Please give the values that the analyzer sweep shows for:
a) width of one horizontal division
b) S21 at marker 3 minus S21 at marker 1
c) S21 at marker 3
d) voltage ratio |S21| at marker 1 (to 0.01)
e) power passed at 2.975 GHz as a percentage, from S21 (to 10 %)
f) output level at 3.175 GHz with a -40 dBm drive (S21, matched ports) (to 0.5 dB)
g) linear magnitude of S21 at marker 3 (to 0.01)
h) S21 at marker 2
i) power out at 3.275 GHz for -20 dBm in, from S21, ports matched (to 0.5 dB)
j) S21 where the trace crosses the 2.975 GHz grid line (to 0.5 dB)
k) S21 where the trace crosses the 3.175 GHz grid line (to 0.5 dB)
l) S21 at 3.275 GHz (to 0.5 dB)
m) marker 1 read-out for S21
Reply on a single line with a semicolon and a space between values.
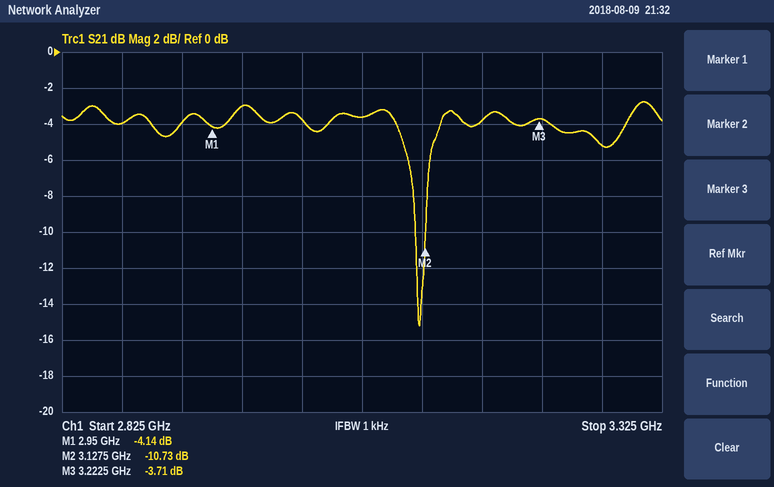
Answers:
50 MHz; 0.43 dB; -3.71 dB; 0.62; 50 %; -44.0 dBm; 0.65; -10.73 dB; -25.0 dBm; -3.0 dB; -4.0 dB; -5.0 dB; -4.14 dB
